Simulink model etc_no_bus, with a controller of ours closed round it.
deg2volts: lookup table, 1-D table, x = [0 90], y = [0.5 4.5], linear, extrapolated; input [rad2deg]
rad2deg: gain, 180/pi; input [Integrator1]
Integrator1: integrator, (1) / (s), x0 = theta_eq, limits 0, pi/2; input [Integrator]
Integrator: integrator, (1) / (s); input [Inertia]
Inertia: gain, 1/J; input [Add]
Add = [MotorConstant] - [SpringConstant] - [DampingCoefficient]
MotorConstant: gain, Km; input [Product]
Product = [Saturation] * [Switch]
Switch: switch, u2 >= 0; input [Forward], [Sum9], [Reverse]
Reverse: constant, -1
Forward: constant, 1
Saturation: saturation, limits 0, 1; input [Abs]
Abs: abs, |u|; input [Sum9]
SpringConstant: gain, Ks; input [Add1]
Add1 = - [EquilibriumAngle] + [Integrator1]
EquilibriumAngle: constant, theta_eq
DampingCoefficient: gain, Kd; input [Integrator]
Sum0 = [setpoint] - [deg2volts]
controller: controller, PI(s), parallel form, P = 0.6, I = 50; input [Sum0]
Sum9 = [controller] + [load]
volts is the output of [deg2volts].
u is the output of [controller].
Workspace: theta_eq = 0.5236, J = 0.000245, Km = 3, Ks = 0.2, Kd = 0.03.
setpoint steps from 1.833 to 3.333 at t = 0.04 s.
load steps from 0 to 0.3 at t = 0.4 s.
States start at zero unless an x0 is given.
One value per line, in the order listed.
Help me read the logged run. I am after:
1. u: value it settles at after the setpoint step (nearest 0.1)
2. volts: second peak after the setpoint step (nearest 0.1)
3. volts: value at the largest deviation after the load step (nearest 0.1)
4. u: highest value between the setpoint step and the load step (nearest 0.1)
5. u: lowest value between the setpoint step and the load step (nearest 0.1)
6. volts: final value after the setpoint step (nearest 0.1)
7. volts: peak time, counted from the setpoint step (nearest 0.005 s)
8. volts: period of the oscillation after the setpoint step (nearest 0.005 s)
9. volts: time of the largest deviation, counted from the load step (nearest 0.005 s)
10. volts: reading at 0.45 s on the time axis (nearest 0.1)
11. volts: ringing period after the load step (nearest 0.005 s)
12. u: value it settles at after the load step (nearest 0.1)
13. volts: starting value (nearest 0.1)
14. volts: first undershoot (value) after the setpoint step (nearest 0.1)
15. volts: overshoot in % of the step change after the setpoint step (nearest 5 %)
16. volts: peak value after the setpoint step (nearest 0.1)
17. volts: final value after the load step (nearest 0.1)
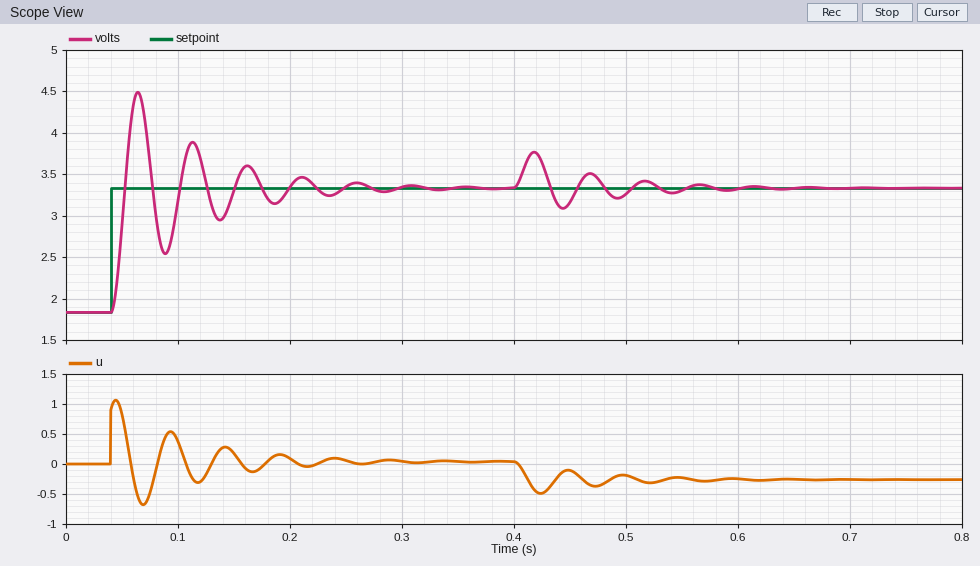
0.0
3.9
3.8
1.1
-0.7
3.3
0.025 s
0.050 s
0.020 s
3.2
0.050 s
-0.3
1.8
2.5
75 %
4.5
3.3
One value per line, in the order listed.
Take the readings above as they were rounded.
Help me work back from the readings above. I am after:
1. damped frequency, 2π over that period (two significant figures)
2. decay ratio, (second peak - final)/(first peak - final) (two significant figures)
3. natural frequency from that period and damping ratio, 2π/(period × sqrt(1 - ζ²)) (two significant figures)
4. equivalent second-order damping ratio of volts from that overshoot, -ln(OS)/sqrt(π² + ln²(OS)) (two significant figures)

130 rad/s
0.50
130 rad/s
0.091
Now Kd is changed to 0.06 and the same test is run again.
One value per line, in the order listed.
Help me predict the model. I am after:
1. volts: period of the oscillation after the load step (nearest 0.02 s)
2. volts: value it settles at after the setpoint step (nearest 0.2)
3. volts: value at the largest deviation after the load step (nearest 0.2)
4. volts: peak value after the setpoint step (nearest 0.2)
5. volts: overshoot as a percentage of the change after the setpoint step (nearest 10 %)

0.08 s
3.4
3.6
4.2
50 %
